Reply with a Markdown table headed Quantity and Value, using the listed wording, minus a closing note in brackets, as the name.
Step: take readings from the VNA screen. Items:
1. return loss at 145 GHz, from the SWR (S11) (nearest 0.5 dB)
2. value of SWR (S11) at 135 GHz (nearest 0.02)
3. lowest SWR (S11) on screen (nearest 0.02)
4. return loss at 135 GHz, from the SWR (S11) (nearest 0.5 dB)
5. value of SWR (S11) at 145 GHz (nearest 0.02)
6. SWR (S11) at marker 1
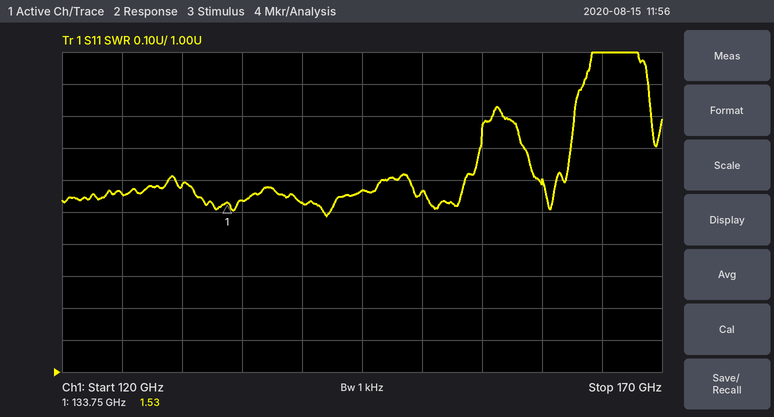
| Quantity | Value |
|---|---|
| return loss at 145 GHz, from the SWR (S11) | 13.0 dB |
| value of SWR (S11) at 135 GHz | 1.54 |
| lowest SWR (S11) on screen | 1.48 |
| return loss at 135 GHz, from the SWR (S11) | 13.5 dB |
| value of SWR (S11) at 145 GHz | 1.56 |
| SWR (S11) at marker 1 | 1.53 |
